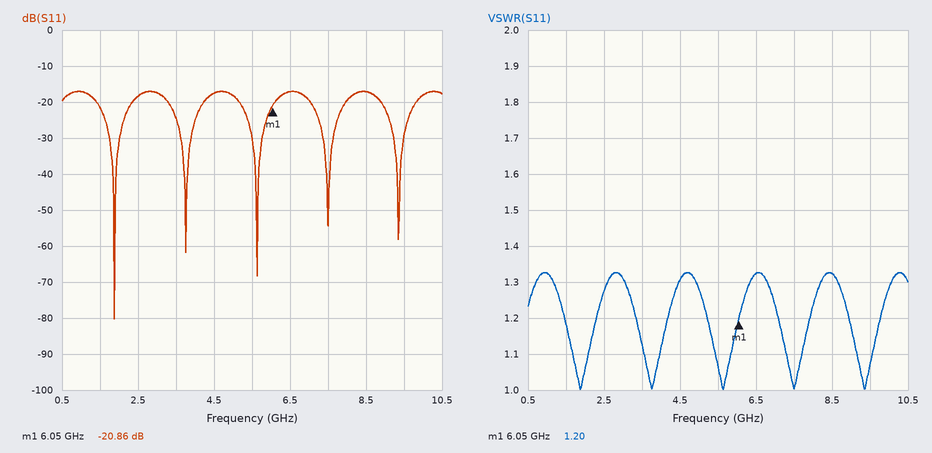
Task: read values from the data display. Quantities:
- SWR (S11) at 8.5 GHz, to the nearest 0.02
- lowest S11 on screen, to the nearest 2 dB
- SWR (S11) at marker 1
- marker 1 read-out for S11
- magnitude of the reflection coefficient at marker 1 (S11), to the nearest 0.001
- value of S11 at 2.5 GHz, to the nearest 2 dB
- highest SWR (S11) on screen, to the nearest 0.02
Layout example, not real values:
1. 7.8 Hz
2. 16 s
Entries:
1. 1.32
2. -80 dB
3. 1.20
4. -20.86 dB
5. 0.091
6. -18 dB
7. 1.32
